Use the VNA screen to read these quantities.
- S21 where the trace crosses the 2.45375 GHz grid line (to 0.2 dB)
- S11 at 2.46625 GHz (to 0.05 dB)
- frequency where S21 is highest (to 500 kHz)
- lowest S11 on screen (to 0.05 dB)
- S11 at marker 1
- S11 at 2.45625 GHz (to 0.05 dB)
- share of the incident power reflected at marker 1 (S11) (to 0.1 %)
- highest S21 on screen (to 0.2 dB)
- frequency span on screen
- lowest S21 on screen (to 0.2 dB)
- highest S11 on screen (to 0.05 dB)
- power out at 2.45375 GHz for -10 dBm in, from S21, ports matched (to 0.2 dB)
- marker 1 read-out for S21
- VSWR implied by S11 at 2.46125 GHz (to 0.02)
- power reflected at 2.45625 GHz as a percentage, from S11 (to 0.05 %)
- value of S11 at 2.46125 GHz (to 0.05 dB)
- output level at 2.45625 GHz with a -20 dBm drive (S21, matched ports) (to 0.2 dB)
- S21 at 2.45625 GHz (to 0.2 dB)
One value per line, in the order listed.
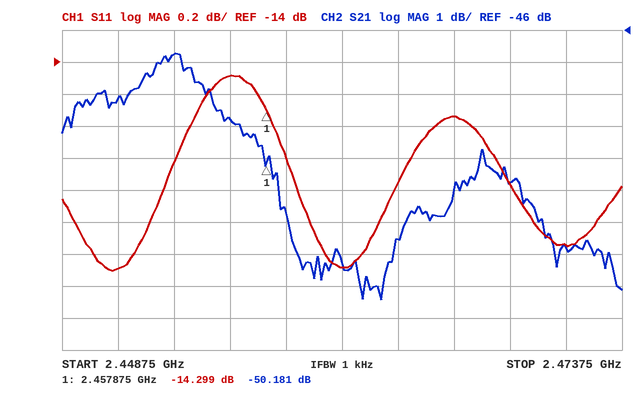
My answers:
-46.8 dB
-14.35 dB
2.4540 GHz
-15.30 dB
-14.299 dB
-14.10 dB
3.7 %
-46.8 dB
25 MHz
-54.4 dB
-14.10 dB
-56.8 dBm
-50.181 dB
1.42
3.90 %
-15.30 dB
-68.8 dBm
-48.8 dB
